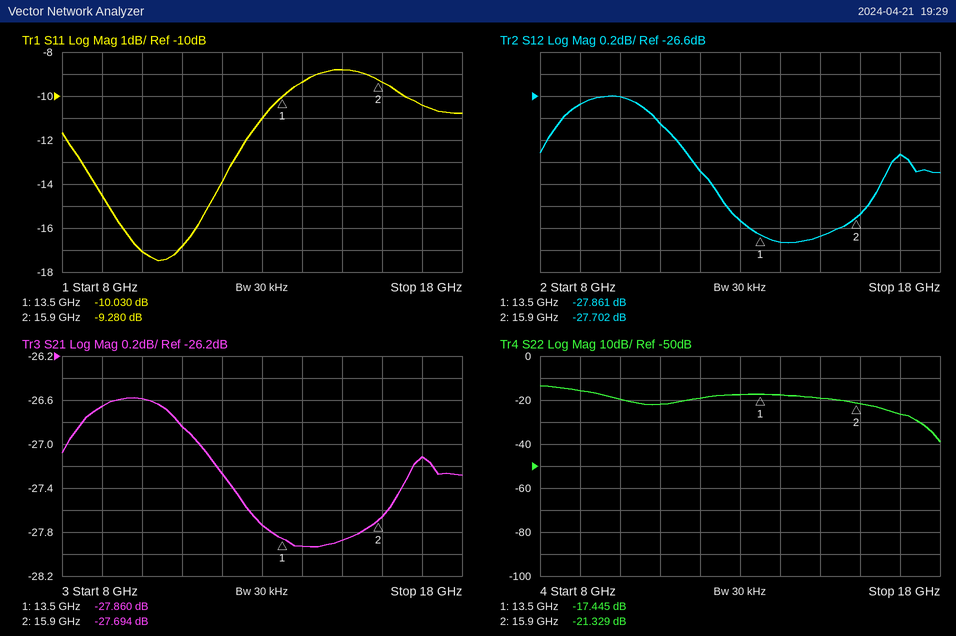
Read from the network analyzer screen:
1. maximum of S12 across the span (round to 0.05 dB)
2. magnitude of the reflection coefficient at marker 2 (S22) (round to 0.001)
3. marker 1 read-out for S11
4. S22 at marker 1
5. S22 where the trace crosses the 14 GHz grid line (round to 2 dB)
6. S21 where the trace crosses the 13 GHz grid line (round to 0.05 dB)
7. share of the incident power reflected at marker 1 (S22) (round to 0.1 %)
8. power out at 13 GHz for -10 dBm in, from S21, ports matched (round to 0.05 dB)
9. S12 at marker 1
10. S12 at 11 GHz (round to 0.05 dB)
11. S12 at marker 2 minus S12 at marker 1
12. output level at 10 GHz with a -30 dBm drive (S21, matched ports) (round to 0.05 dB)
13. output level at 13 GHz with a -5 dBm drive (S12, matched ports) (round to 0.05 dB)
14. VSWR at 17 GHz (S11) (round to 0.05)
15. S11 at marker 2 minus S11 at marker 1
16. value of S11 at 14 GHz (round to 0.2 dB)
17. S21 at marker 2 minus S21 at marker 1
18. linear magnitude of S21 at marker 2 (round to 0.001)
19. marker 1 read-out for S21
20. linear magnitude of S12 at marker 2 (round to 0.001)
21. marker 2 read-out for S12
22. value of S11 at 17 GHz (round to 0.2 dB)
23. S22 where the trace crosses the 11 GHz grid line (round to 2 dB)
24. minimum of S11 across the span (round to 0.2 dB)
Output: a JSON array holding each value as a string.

["-26.60 dB", "0.086", "-10.030 dB", "-17.445 dB", "-18 dB", "-27.75 dB", "1.8 %", "-37.75 dBm", "-27.861 dB", "-26.85 dB", "0.159 dB", "-56.60 dBm", "-32.75 dBm", "1.85", "0.750 dB", "-9.4 dB", "0.166 dB", "0.041", "-27.860 dB", "0.041", "-27.702 dB", "-10.4 dB", "-22 dB", "-17.4 dB"]
